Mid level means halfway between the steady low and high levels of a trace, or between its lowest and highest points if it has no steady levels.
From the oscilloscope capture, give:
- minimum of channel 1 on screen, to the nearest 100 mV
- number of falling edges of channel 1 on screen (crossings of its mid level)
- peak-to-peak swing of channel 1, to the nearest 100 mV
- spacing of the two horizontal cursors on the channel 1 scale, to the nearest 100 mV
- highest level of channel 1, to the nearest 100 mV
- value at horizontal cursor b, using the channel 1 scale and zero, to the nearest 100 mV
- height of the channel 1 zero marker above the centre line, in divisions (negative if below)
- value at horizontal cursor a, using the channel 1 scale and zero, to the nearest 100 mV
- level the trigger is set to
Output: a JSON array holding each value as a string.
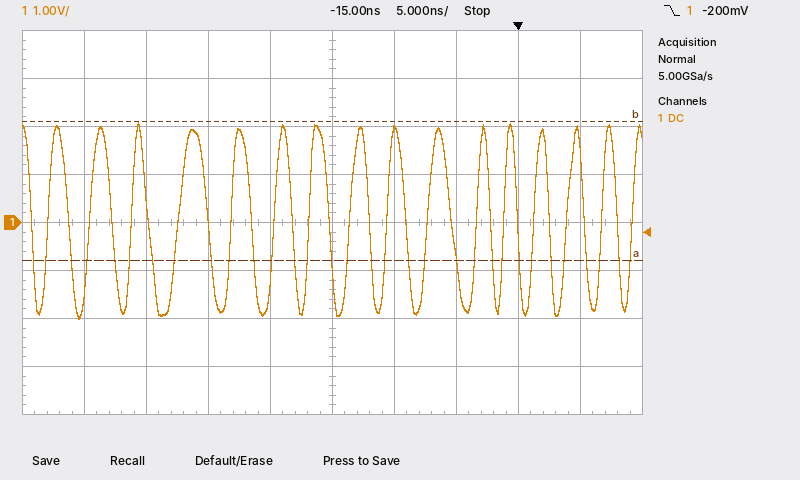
["-2.0 V", "16", "4.1 V", "2.9 V", "2.1 V", "2.1 V", "0.0 div", "-800 mV", "-200 mV"]
